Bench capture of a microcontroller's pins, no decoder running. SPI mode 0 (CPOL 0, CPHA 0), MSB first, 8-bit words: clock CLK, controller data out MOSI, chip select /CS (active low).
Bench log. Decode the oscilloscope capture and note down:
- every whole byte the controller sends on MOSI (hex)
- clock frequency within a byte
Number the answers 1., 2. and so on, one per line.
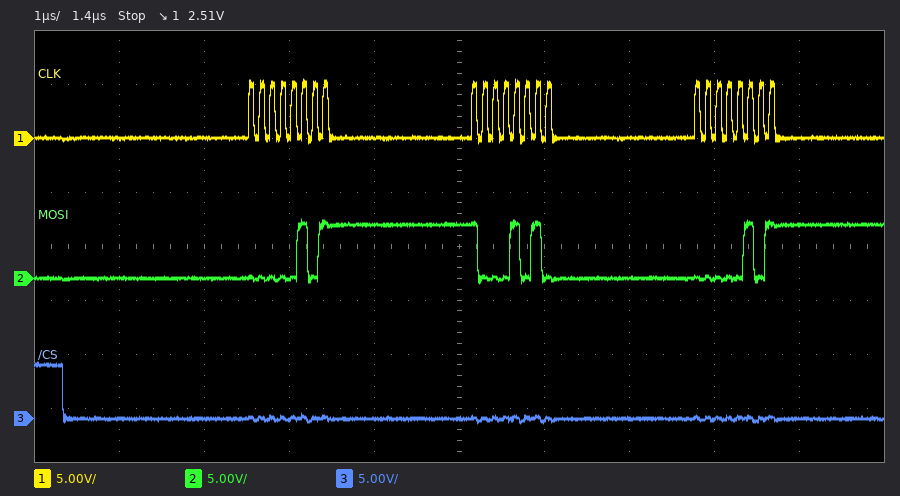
1. 05 8A 05
2. 8 MHz
